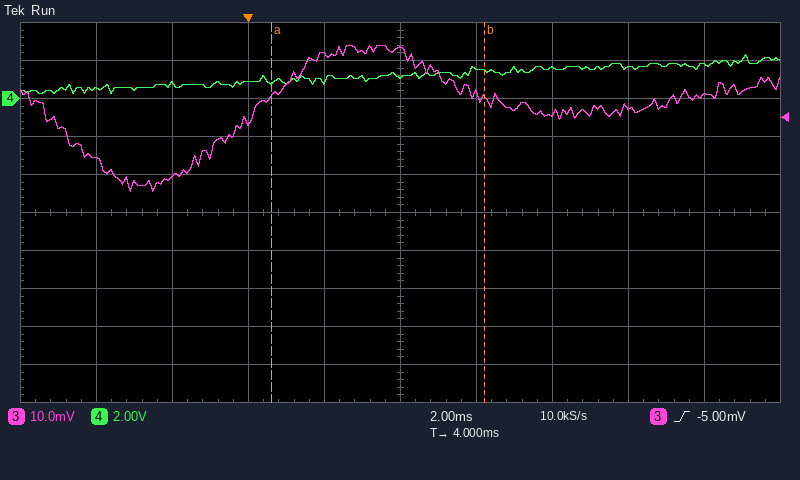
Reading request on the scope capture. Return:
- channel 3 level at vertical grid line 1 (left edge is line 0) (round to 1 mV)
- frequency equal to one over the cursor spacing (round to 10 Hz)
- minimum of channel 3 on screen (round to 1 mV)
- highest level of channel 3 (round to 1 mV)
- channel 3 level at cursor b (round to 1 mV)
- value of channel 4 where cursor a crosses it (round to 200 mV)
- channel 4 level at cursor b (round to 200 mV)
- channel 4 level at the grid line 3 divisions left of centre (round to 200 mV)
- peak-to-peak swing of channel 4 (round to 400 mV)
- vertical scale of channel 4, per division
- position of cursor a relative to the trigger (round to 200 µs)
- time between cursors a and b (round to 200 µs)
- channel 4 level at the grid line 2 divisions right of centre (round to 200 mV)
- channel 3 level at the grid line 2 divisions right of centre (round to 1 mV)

-16 mV
180 Hz
-24 mV
14 mV
0 mV
800 mV
1.4 V
800 mV
2.0 V
2 V
+600 µs
5.6 ms
1.6 V
-4 mV
